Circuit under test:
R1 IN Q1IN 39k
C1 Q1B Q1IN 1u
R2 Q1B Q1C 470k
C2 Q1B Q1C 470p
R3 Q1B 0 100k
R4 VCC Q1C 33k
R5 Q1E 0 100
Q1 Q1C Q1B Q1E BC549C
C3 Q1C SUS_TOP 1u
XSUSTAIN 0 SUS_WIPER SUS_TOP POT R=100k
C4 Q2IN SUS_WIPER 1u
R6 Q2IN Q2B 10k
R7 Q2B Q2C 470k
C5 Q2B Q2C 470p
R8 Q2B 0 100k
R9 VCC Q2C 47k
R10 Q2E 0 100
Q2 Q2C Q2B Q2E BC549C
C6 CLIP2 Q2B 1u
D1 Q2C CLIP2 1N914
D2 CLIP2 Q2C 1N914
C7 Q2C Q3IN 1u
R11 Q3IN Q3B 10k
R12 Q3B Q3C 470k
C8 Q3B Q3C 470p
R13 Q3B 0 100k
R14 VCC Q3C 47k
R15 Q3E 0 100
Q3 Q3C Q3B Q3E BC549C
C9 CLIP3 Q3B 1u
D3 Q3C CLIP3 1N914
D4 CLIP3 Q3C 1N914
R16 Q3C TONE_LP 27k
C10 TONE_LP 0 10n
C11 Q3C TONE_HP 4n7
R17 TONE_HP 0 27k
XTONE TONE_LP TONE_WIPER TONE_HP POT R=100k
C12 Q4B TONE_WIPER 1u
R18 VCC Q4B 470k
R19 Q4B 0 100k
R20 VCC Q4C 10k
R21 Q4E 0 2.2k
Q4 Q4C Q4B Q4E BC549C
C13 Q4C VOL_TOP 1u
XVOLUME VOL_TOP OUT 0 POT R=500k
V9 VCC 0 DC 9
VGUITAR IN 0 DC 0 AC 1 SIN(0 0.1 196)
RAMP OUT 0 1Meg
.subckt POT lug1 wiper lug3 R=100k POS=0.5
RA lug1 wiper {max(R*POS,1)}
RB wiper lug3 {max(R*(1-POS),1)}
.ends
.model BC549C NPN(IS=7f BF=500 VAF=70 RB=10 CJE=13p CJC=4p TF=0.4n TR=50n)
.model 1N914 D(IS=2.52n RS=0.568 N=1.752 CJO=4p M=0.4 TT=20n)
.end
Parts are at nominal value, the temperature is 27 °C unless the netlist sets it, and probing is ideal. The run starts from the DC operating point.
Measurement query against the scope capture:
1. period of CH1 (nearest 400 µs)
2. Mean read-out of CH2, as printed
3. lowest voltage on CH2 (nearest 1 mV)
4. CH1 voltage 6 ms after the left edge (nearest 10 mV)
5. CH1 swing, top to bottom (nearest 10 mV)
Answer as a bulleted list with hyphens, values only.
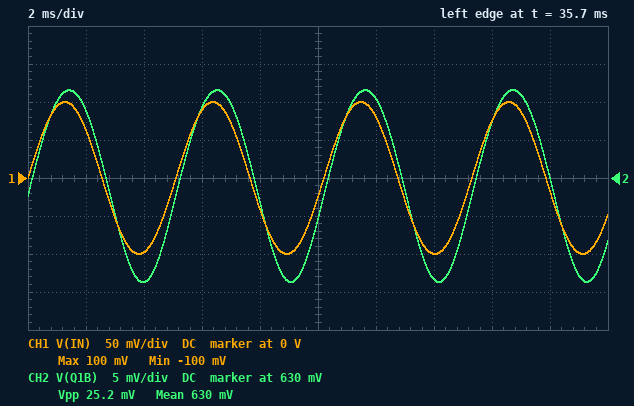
- 5.2 ms
- 630 mV
- 616 mV
- 90 mV
- 200 mV
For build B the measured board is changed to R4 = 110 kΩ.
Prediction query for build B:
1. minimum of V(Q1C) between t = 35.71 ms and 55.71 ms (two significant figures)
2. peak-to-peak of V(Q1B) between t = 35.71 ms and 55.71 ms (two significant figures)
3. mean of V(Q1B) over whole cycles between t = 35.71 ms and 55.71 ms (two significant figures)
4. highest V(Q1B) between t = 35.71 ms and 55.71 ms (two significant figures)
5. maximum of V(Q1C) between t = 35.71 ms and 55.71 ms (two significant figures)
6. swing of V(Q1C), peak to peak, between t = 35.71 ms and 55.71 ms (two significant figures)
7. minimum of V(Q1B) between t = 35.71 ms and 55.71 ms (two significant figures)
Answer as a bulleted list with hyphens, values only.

- 2.5 V
- 35 mV
- 590 mV
- 600 mV
- 4.2 V
- 1.7 V
- 570 mV
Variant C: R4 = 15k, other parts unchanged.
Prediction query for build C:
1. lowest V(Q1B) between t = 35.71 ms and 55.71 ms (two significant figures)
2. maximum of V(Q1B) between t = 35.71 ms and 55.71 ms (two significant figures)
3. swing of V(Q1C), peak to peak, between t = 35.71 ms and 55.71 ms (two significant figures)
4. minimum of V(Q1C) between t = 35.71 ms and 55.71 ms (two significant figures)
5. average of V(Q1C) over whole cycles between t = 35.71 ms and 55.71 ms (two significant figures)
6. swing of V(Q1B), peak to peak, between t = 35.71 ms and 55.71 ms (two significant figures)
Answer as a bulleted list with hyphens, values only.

- 650 mV
- 680 mV
- 1.7 V
- 3.2 V
- 4.1 V
- 28 mV
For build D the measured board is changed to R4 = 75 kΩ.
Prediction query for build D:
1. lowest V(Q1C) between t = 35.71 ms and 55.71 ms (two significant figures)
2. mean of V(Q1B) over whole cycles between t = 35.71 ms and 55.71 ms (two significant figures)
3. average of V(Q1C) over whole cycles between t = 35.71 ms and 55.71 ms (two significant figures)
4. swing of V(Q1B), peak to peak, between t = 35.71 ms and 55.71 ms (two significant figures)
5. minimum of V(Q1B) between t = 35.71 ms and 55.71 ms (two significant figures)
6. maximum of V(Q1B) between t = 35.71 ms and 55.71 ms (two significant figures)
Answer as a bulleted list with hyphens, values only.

- 2.6 V
- 600 mV
- 3.5 V
- 30 mV
- 580 mV
- 610 mV
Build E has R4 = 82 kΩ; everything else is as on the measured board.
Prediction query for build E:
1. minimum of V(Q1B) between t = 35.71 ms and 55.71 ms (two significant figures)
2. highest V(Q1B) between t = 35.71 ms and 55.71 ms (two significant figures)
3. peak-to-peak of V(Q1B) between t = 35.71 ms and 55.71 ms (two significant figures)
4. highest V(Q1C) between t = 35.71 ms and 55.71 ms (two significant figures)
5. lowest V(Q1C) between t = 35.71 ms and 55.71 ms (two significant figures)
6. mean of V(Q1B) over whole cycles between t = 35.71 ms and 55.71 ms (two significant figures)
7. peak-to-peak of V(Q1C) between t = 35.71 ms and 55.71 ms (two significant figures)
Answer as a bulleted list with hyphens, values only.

- 580 mV
- 610 mV
- 31 mV
- 4.3 V
- 2.6 V
- 600 mV
- 1.8 V
